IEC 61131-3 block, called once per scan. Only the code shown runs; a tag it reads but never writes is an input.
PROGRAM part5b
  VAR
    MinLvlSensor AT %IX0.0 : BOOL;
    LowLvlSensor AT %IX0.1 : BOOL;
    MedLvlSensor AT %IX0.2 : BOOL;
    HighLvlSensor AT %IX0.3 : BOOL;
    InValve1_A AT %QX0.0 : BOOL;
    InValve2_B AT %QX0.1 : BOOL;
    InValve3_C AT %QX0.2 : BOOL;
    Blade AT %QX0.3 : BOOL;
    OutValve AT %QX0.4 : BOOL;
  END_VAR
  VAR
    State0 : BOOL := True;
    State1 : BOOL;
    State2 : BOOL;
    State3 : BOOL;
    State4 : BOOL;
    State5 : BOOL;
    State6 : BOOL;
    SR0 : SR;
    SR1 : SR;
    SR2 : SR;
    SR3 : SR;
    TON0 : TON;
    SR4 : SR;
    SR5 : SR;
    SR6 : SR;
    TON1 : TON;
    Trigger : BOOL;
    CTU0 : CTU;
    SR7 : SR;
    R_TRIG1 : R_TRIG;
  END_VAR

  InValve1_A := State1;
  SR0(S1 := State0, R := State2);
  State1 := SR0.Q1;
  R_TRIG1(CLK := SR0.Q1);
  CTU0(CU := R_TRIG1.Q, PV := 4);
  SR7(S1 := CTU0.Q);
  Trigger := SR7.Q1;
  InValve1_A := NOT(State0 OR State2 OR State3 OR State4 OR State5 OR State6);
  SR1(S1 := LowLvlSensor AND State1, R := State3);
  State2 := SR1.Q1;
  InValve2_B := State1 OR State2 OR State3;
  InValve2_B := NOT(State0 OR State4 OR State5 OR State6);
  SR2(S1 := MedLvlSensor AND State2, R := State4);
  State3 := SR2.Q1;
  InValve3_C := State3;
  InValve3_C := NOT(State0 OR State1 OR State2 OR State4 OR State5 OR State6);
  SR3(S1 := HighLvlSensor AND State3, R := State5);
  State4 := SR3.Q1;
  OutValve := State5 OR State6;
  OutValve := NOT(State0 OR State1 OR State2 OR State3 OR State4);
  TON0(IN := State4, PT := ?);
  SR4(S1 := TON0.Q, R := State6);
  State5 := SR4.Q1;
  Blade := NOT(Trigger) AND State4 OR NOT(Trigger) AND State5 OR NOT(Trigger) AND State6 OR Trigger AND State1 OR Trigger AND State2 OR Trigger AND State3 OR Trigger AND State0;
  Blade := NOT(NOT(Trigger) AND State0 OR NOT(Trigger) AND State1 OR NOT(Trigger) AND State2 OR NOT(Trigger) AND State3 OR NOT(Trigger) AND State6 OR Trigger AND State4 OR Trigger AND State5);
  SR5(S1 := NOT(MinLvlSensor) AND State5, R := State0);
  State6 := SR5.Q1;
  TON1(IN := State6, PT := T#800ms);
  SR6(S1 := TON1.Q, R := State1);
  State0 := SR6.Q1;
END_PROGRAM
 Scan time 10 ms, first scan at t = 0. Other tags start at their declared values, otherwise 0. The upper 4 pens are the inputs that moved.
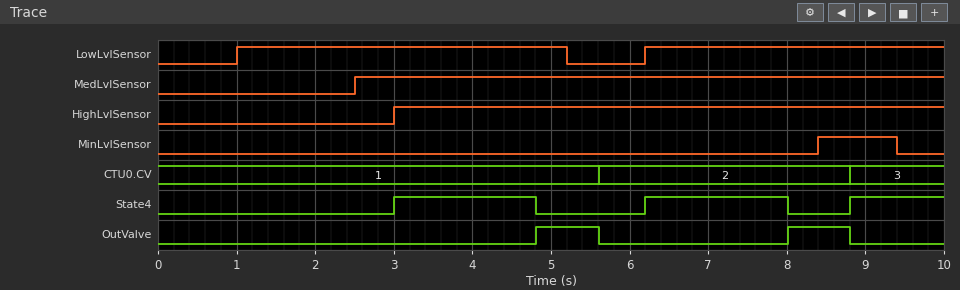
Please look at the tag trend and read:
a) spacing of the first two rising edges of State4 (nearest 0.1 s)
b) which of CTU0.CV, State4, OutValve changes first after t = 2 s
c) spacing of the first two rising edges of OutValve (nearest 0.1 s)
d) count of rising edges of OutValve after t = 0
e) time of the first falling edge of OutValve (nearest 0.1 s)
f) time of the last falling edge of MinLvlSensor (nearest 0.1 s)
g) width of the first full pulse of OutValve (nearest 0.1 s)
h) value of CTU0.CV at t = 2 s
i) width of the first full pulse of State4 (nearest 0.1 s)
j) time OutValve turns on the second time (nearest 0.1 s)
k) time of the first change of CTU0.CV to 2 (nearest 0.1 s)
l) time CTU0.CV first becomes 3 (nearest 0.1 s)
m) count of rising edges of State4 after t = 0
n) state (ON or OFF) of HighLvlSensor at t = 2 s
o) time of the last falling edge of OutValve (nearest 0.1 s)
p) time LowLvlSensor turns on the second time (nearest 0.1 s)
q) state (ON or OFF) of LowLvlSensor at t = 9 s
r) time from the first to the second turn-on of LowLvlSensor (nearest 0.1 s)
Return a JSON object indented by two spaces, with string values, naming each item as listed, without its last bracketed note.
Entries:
{
  "spacing of the first two rising edges of State4": "3.2 s",
  "which of CTU0.CV, State4, OutValve changes first after t = 2 s": "State4",
  "spacing of the first two rising edges of OutValve": "3.2 s",
  "count of rising edges of OutValve after t = 0": "2",
  "time of the first falling edge of OutValve": "5.6 s",
  "time of the last falling edge of MinLvlSensor": "9.4 s",
  "width of the first full pulse of OutValve": "0.8 s",
  "value of CTU0.CV at t = 2 s": "1",
  "width of the first full pulse of State4": "1.8 s",
  "time OutValve turns on the second time": "8.0 s",
  "time of the first change of CTU0.CV to 2": "5.6 s",
  "time CTU0.CV first becomes 3": "8.8 s",
  "count of rising edges of State4 after t = 0": "3",
  "state (ON or OFF) of HighLvlSensor at t = 2 s": "OFF",
  "time of the last falling edge of OutValve": "8.8 s",
  "time LowLvlSensor turns on the second time": "6.2 s",
  "state (ON or OFF) of LowLvlSensor at t = 9 s": "ON",
  "time from the first to the second turn-on of LowLvlSensor": "5.2 s"
}
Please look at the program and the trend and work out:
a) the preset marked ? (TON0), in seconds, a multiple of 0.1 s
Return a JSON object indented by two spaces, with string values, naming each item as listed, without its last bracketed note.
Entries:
{
  "the preset marked ? (TON0), in seconds, a multiple of 0.1 s": "1.8 s"
}
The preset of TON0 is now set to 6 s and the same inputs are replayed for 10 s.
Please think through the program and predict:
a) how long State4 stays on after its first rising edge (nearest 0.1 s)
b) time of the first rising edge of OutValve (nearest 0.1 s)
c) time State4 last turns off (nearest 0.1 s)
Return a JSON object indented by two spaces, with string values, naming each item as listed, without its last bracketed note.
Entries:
{
  "how long State4 stays on after its first rising edge": "6.0 s",
  "time of the first rising edge of OutValve": "9.0 s",
  "time State4 last turns off": "9.0 s"
}
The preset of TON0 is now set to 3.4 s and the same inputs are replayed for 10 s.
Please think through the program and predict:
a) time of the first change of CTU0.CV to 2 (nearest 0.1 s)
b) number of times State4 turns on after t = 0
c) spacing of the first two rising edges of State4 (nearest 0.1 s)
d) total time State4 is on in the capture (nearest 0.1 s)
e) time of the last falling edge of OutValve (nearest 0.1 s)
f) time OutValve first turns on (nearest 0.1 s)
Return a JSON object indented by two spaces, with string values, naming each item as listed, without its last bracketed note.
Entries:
{
  "time of the first change of CTU0.CV to 2": "7.2 s",
  "number of times State4 turns on after t = 0": "2",
  "spacing of the first two rising edges of State4": "4.2 s",
  "total time State4 is on in the capture": "6.2 s",
  "time of the last falling edge of OutValve": "7.2 s",
  "time OutValve first turns on": "6.4 s"
}
